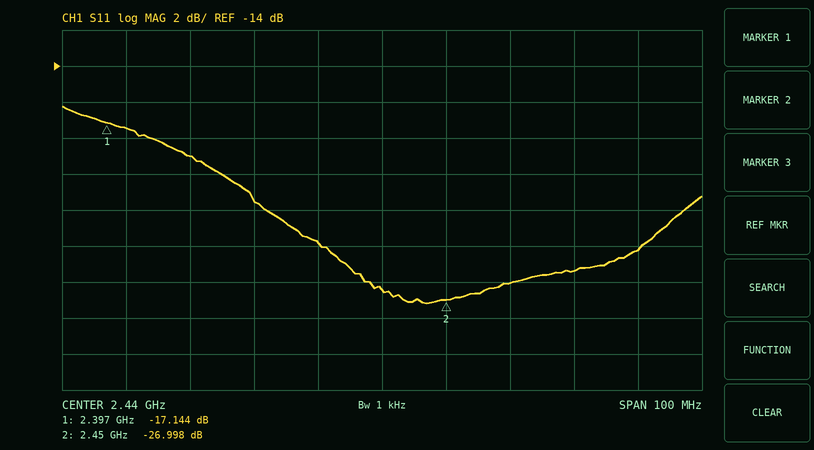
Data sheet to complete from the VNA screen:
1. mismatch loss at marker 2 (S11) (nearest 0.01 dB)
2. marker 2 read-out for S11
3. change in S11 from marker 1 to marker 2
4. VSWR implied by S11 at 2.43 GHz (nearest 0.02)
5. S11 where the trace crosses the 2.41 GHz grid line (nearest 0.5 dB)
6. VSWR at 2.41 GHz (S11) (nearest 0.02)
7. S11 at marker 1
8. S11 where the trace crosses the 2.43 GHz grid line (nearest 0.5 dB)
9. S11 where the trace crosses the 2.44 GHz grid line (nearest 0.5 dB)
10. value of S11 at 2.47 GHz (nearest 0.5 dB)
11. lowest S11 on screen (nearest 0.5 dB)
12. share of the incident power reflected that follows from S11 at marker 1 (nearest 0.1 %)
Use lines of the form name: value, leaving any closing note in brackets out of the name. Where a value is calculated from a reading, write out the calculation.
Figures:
mismatch loss at marker 2 (S11): −10 log10(1 − 10^(-26.998/10)) ≈ 0.01 dB
marker 2 read-out for S11: -26.998 dB
change in S11 from marker 1 to marker 2: -26.998 − (-17.144) = -9.854 dB
VSWR implied by S11 at 2.43 GHz: |Γ| = 10^(-24/20) = 0.0631; VSWR = (1 + 0.0631)/(1 − 0.0631) ≈ 1.13, so 1.14 to the nearest 0.02
S11 where the trace crosses the 2.41 GHz grid line: -19.0 dB
VSWR at 2.41 GHz (S11): |Γ| = 10^(-19/20) = 0.1122; VSWR = (1 + 0.1122)/(1 − 0.1122) ≈ 1.25, so 1.26 to the nearest 0.02
S11 at marker 1: -17.144 dB
S11 where the trace crosses the 2.43 GHz grid line: -24.0 dB
S11 where the trace crosses the 2.44 GHz grid line: -26.5 dB
value of S11 at 2.47 GHz: -25.5 dB
lowest S11 on screen: -27.0 dB
share of the incident power reflected that follows from S11 at marker 1: 10^(-17.144/10) ≈ 1.9 %
